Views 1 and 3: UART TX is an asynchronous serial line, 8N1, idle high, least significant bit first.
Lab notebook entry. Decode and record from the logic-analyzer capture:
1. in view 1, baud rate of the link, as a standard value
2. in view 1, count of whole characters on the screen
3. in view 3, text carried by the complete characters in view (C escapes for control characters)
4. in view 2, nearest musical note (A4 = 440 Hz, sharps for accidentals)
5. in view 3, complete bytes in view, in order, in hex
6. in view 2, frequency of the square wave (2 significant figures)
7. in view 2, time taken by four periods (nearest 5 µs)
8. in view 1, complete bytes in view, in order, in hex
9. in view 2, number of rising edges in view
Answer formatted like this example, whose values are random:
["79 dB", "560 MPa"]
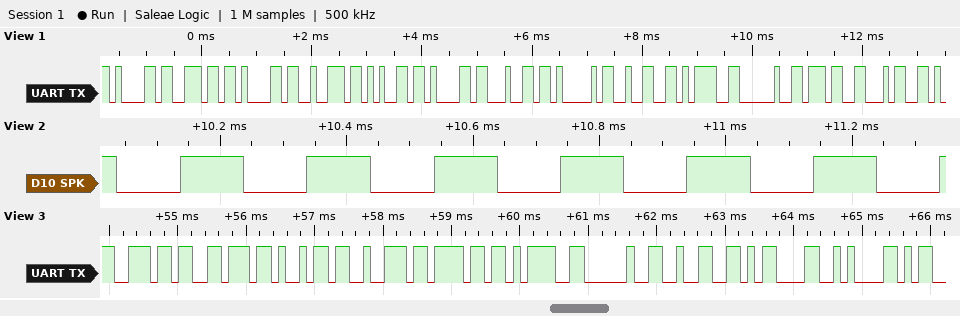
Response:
["9600 baud", "13", "\"nviro= 2\\r\\n\"", "D#8", "0x6E 0x76 0x69 0x72 0x6F 0x3D 0x20 0x32 0x0D 0x0A", "5.0 kHz", "800 µs", "61 6E 61 72 65 61 64 41 32 3D 20 37 34", "7"]
